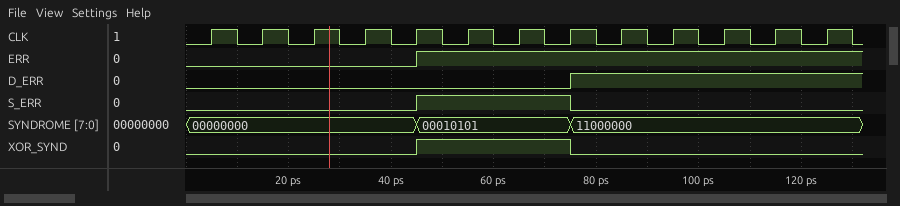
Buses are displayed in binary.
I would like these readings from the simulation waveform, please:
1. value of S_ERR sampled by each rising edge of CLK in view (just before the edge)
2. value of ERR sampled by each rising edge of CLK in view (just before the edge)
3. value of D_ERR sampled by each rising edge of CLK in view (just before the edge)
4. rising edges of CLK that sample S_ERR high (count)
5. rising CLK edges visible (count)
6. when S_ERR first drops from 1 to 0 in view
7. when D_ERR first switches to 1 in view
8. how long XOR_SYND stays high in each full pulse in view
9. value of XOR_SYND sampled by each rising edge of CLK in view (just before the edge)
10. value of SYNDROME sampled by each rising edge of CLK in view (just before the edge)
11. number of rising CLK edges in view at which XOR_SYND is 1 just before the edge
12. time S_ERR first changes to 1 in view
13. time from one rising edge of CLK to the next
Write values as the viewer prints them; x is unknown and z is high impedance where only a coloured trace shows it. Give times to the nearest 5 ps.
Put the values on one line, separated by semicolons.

0 0 0 0 0 1 1 1 0 0 0 0 0; 0 0 0 0 0 1 1 1 1 1 1 1 1; 0 0 0 0 0 0 0 0 1 1 1 1 1; 3; 13; 75 ps; 75 ps; 30 ps; 0 0 0 0 0 1 1 1 0 0 0 0 0; 00000000, 00000000, 00000000, 00000000, 00000000, 00010101, 00010101, 00010101, 11000000, 11000000, 11000000, 11000000, 11000000; 3; 45 ps; 10 ps
